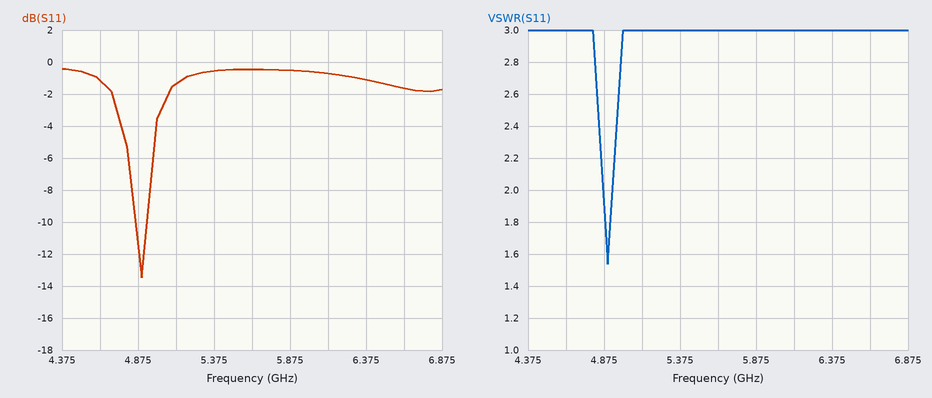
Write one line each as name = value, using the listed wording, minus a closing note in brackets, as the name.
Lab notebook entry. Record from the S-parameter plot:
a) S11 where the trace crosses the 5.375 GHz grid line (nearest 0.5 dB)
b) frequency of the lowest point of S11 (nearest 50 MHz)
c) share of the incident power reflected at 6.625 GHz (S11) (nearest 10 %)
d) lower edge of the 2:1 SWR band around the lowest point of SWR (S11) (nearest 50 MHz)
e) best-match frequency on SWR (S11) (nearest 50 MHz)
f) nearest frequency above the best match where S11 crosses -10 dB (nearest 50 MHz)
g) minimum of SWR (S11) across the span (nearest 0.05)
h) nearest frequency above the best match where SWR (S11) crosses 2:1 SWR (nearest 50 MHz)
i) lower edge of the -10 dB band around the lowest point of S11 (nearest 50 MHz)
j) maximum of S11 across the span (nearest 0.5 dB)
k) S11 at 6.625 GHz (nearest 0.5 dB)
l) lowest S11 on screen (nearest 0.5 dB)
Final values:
S11 where the trace crosses the 5.375 GHz grid line = -0.5 dB
frequency of the lowest point of S11 = 4.90 GHz
share of the incident power reflected at 6.625 GHz (S11) = 70 %
lower edge of the 2:1 SWR band around the lowest point of SWR (S11) = 4.85 GHz
best-match frequency on SWR (S11) = 4.90 GHz
nearest frequency above the best match where S11 crosses -10 dB = 4.95 GHz
minimum of SWR (S11) across the span = 1.55
nearest frequency above the best match where SWR (S11) crosses 2:1 SWR = 4.95 GHz
lower edge of the -10 dB band around the lowest point of S11 = 4.85 GHz
maximum of S11 across the span = -0.5 dB
S11 at 6.625 GHz = -1.5 dB
lowest S11 on screen = -13.5 dB
